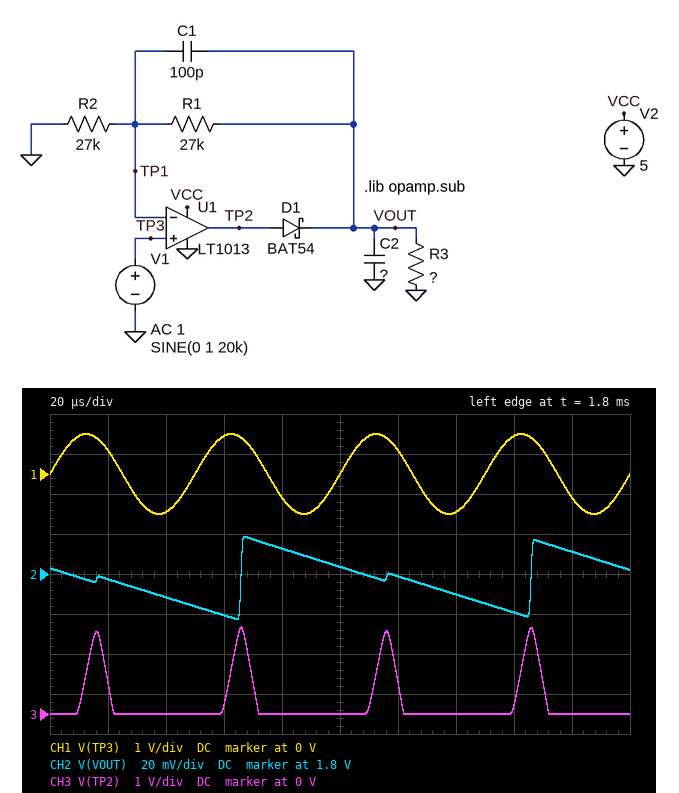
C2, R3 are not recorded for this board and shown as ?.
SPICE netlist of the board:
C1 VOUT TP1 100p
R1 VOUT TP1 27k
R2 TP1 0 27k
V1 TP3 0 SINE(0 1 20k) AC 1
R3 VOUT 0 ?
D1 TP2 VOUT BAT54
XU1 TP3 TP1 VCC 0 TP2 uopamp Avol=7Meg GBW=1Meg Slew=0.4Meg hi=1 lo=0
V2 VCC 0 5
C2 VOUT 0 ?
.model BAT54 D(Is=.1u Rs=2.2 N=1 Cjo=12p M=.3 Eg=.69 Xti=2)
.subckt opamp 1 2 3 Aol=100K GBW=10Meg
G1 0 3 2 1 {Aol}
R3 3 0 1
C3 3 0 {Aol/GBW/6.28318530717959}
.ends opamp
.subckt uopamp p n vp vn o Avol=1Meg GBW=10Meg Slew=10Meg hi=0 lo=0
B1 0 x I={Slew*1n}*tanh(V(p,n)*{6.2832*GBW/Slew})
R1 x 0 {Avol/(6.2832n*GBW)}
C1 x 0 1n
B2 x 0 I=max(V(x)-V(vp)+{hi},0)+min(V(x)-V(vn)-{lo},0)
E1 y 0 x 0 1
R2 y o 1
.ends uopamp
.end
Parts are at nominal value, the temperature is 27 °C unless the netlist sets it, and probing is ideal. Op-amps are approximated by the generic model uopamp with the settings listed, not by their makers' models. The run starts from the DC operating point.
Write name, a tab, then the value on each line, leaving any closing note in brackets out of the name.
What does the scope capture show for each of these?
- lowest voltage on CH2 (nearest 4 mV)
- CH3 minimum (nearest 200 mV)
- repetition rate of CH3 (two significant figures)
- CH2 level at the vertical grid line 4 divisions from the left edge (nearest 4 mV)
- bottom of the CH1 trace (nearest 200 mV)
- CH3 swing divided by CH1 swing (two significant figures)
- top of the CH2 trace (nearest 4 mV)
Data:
lowest voltage on CH2	1.776 V
CH3 minimum	0 V
repetition rate of CH3	20 kHz
CH2 level at the vertical grid line 4 divisions from the left edge	1.812 V
bottom of the CH1 trace	-1.0 V
CH3 swing divided by CH1 swing	1.1
top of the CH2 trace	1.820 V
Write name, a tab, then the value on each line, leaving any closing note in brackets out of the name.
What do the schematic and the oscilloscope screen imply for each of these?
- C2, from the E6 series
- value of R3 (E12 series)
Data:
C2, from the E6 series	470 nF
value of R3	10 kΩ
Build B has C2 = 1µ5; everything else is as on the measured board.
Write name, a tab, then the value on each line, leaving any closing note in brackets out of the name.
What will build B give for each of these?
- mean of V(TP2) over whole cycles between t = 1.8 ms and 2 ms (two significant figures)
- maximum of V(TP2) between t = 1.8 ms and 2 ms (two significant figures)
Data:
mean of V(TP2) over whole cycles between t = 1.8 ms and 2 ms	300 mV
maximum of V(TP2) between t = 1.8 ms and 2 ms	2.1 V
